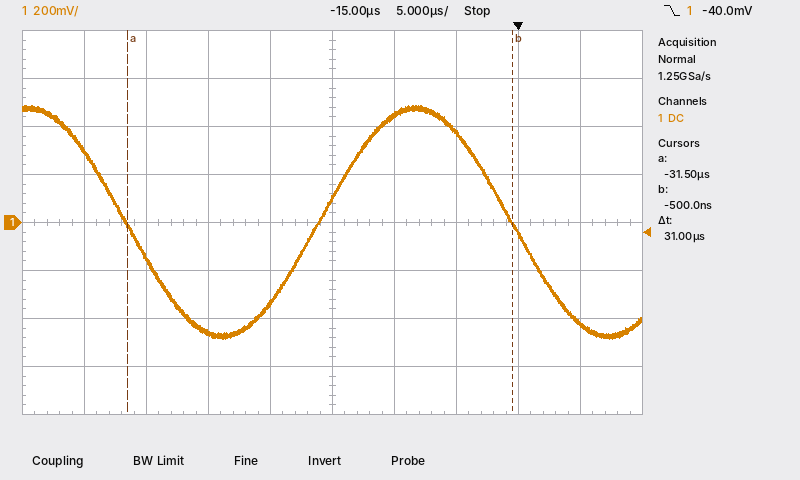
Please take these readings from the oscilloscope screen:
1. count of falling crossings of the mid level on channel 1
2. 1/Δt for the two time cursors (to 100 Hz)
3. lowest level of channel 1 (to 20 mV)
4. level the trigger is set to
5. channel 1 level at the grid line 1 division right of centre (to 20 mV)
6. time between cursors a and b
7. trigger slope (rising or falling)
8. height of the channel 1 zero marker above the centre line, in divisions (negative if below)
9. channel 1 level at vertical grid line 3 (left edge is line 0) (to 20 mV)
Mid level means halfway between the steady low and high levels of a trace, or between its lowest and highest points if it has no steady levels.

2
32.3 kHz
-480 mV
-40.0 mV
440 mV
31 µs
falling
0.0 div
-460 mV
